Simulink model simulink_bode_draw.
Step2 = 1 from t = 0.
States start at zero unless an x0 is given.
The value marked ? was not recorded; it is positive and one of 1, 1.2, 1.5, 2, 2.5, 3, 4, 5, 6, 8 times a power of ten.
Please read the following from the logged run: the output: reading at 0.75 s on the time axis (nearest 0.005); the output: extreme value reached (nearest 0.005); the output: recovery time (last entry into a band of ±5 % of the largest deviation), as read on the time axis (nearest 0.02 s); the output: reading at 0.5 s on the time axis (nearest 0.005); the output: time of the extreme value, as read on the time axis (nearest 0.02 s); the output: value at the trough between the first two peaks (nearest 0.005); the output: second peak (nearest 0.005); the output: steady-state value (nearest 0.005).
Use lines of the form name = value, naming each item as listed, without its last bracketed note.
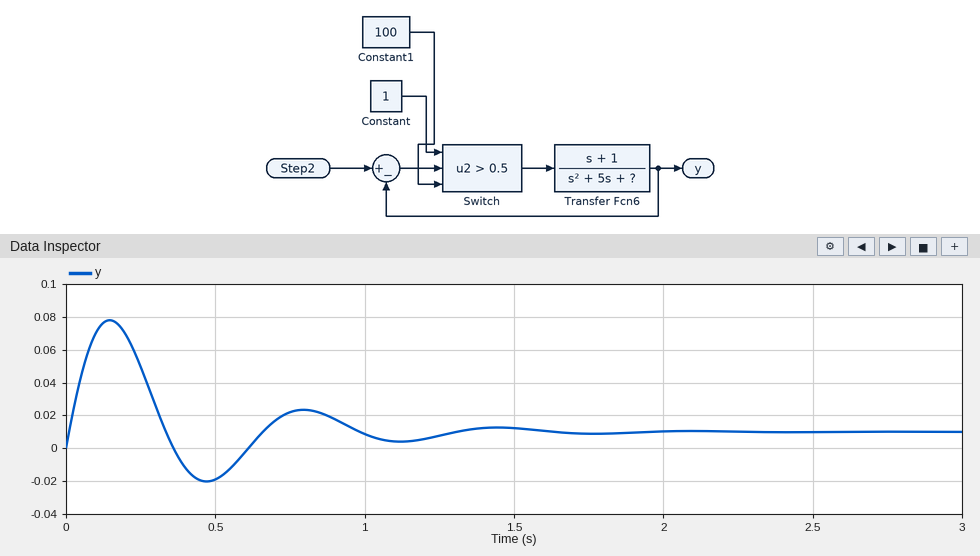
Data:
the output: reading at 0.75 s on the time axis = 0.020
the output: extreme value reached = 0.080
the output: recovery time (last entry into a band of ±5 % of the largest deviation), as read on the time axis = 1.22 s
the output: reading at 0.5 s on the time axis = -0.020
the output: time of the extreme value, as read on the time axis = 0.14 s
the output: value at the trough between the first two peaks = -0.020
the output: second peak = 0.025
the output: steady-state value = 0.010
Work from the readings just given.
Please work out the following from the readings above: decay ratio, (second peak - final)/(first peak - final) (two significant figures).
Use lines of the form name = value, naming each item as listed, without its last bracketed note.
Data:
decay ratio, (second peak - final)/(first peak - final) = 0.21
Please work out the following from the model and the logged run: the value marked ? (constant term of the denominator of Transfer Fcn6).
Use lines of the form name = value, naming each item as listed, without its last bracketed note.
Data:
the value marked ? = 100
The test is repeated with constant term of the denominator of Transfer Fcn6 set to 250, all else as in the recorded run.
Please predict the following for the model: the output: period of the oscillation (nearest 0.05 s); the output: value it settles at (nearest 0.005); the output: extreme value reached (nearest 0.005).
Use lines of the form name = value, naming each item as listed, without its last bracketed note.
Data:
the output: period of the oscillation = 0.40 s
the output: value it settles at = 0.005
the output: extreme value reached = 0.055
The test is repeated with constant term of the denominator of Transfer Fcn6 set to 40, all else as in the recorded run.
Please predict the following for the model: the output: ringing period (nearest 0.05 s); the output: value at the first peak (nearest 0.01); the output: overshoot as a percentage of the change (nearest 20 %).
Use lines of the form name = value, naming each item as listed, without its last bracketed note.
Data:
the output: ringing period = 1.10 s
the output: value at the first peak = 0.11
the output: overshoot as a percentage of the change = 340 %
